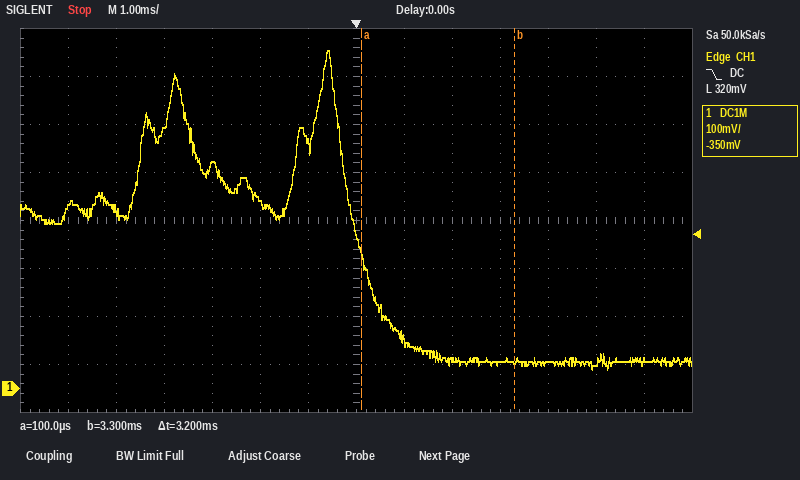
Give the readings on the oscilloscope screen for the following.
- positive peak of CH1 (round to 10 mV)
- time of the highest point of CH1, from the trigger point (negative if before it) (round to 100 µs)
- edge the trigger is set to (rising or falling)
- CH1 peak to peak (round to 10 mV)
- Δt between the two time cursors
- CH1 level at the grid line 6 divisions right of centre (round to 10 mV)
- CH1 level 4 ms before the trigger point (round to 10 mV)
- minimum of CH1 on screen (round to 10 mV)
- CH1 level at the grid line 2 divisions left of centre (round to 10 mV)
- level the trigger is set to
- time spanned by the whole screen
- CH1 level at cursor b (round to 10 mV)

700 mV
-600 µs
falling
660 mV
3.2 ms
60 mV
540 mV
40 mV
390 mV
320 mV
14 ms
60 mV
